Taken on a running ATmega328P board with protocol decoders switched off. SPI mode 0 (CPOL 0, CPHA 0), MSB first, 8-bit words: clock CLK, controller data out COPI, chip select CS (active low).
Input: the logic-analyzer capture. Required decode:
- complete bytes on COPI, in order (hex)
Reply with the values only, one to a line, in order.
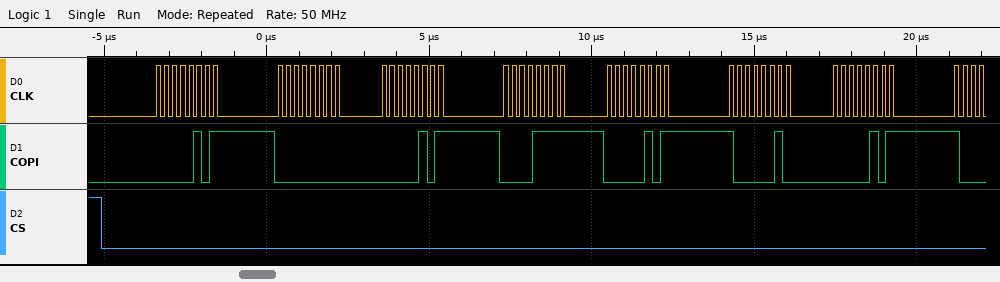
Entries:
05 00 05 0F 05 82 05
